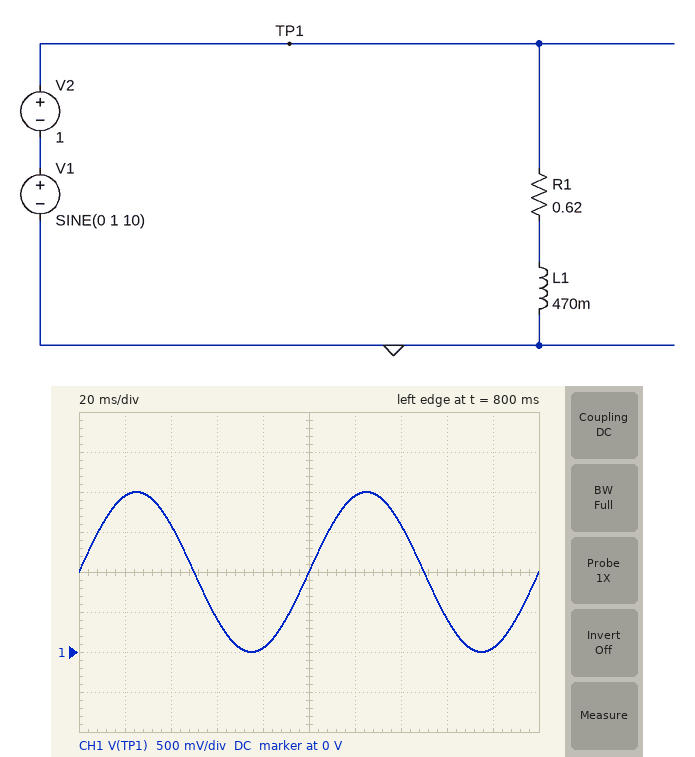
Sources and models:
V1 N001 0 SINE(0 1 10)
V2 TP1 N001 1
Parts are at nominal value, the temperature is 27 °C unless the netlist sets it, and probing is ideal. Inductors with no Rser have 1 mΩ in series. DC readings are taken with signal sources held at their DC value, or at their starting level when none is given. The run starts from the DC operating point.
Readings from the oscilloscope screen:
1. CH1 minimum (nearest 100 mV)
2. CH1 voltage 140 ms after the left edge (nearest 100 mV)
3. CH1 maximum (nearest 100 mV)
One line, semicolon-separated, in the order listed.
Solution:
0 V; 1.6 V; 2.0 V
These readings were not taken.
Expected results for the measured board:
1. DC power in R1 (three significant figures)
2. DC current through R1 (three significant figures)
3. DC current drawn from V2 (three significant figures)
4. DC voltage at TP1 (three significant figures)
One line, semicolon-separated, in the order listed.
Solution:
1.61 W; 1.61 A; 1.61 A; 1.00 V
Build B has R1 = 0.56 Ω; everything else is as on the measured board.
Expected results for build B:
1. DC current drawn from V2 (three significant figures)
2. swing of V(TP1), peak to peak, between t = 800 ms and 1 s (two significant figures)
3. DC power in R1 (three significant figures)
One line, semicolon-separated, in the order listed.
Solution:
1.78 A; 2.0 V; 1.78 W
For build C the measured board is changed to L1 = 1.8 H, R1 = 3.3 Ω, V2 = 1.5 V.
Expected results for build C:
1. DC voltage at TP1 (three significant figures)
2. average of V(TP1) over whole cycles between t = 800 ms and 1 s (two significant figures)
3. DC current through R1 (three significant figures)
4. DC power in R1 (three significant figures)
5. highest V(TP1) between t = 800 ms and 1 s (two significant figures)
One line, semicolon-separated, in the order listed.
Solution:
1.50 V; 1.5 V; 454 mA; 681 mW; 2.5 V
